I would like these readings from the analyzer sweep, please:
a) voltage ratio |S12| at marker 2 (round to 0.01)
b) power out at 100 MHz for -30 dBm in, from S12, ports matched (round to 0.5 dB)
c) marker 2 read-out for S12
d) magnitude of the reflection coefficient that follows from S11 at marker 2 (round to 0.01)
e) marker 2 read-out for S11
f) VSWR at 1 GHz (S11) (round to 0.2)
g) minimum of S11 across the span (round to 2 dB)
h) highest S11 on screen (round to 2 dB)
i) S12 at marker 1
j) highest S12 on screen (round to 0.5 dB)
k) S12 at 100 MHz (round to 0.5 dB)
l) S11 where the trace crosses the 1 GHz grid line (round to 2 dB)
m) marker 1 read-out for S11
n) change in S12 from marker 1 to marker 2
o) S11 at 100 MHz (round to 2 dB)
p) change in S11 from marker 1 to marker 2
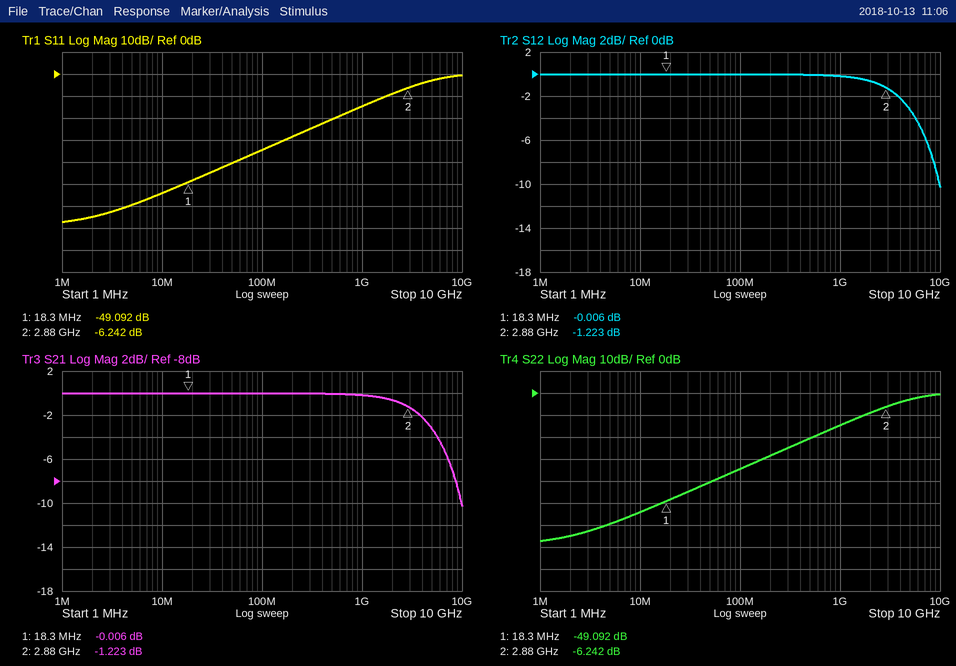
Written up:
0.87
-30.0 dBm
-1.223 dB
0.49
-6.242 dB
1.4
-68 dB
0 dB
-0.006 dB
0.0 dB
0.0 dB
-14 dB
-49.092 dB
-1.217 dB
-34 dB
42.850 dB
